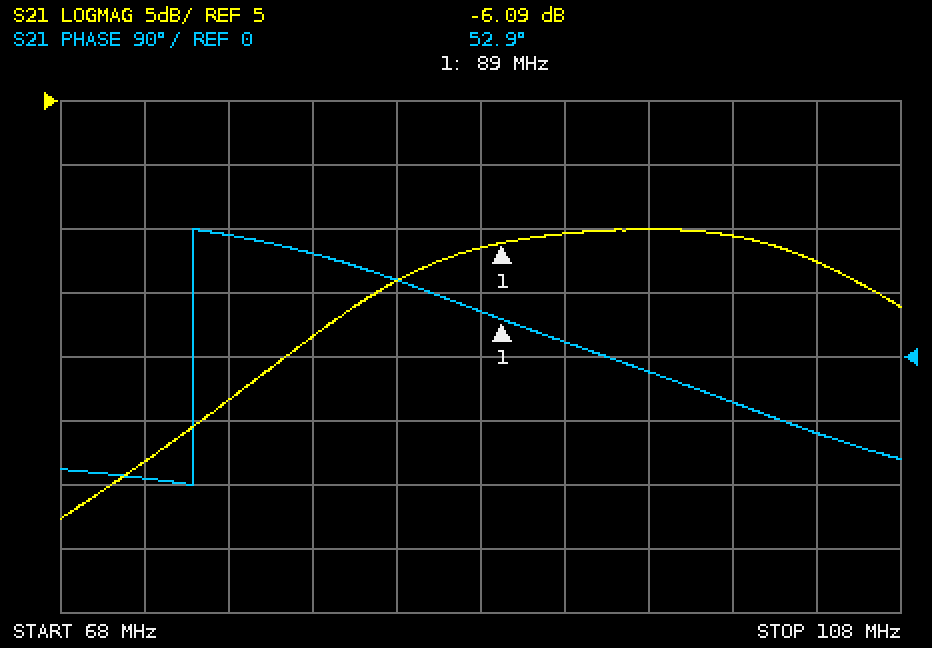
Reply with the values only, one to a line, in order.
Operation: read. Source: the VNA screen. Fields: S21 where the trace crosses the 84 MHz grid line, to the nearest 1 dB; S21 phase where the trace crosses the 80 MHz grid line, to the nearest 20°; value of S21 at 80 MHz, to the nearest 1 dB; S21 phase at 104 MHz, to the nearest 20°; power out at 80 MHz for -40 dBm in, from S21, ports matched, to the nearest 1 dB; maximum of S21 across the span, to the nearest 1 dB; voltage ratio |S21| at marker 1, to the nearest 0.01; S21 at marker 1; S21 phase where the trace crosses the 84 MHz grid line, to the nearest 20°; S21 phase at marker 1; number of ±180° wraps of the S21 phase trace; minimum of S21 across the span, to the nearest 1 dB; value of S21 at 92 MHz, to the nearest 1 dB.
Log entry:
-9 dB
140°
-13 dB
-100°
-53 dBm
-5 dB
0.50
-6.09 dB
100°
52.9°
1
-28 dB
-5 dB
